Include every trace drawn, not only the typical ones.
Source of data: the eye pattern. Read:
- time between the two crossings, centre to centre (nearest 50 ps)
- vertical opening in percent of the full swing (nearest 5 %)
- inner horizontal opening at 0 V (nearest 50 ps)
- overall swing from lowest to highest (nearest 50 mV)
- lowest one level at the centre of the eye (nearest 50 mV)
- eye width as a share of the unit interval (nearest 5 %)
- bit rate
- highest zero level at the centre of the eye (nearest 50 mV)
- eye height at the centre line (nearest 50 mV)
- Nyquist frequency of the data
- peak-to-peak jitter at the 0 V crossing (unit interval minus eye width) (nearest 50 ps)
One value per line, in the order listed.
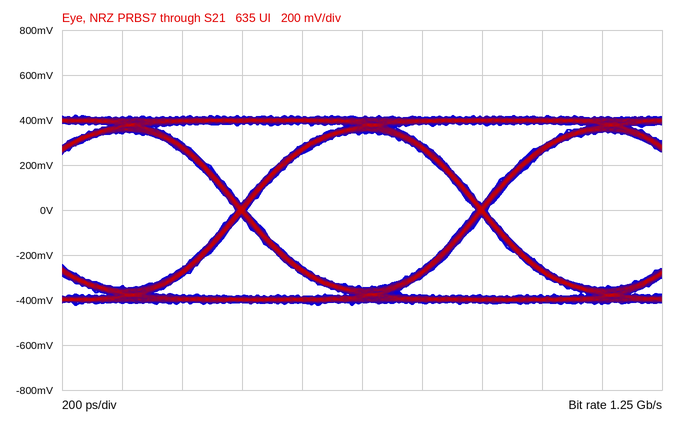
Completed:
800 ps
80 %
750 ps
850 mV
350 mV
95 %
1.25 Gb/s
-350 mV
700 mV
625 MHz
50 ps
